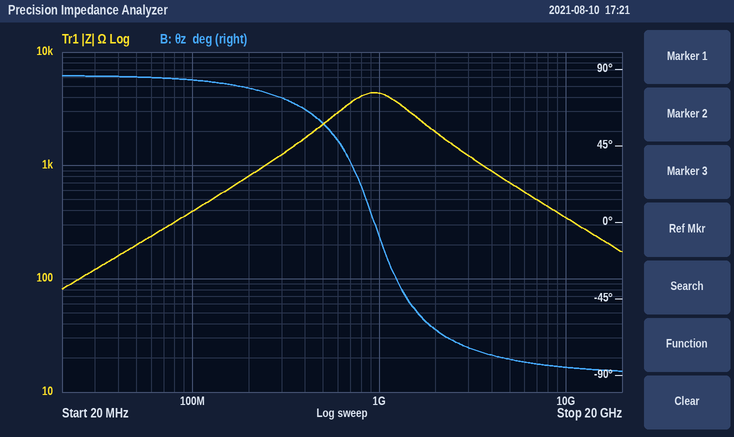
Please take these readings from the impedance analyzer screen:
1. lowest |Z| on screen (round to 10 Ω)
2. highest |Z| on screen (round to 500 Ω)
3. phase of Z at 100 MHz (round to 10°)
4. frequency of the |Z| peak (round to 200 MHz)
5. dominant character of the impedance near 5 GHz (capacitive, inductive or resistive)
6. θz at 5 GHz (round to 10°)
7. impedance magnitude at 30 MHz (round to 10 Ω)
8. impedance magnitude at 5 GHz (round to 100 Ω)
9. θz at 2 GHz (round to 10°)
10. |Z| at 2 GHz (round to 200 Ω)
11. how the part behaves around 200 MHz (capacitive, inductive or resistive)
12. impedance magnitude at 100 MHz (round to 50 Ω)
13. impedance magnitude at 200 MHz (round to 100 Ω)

80 Ω
4.5 kΩ
80°
1.0 GHz
capacitive
-80°
120 Ω
700 Ω
-60°
2.0 kΩ
inductive
400 Ω
800 Ω
